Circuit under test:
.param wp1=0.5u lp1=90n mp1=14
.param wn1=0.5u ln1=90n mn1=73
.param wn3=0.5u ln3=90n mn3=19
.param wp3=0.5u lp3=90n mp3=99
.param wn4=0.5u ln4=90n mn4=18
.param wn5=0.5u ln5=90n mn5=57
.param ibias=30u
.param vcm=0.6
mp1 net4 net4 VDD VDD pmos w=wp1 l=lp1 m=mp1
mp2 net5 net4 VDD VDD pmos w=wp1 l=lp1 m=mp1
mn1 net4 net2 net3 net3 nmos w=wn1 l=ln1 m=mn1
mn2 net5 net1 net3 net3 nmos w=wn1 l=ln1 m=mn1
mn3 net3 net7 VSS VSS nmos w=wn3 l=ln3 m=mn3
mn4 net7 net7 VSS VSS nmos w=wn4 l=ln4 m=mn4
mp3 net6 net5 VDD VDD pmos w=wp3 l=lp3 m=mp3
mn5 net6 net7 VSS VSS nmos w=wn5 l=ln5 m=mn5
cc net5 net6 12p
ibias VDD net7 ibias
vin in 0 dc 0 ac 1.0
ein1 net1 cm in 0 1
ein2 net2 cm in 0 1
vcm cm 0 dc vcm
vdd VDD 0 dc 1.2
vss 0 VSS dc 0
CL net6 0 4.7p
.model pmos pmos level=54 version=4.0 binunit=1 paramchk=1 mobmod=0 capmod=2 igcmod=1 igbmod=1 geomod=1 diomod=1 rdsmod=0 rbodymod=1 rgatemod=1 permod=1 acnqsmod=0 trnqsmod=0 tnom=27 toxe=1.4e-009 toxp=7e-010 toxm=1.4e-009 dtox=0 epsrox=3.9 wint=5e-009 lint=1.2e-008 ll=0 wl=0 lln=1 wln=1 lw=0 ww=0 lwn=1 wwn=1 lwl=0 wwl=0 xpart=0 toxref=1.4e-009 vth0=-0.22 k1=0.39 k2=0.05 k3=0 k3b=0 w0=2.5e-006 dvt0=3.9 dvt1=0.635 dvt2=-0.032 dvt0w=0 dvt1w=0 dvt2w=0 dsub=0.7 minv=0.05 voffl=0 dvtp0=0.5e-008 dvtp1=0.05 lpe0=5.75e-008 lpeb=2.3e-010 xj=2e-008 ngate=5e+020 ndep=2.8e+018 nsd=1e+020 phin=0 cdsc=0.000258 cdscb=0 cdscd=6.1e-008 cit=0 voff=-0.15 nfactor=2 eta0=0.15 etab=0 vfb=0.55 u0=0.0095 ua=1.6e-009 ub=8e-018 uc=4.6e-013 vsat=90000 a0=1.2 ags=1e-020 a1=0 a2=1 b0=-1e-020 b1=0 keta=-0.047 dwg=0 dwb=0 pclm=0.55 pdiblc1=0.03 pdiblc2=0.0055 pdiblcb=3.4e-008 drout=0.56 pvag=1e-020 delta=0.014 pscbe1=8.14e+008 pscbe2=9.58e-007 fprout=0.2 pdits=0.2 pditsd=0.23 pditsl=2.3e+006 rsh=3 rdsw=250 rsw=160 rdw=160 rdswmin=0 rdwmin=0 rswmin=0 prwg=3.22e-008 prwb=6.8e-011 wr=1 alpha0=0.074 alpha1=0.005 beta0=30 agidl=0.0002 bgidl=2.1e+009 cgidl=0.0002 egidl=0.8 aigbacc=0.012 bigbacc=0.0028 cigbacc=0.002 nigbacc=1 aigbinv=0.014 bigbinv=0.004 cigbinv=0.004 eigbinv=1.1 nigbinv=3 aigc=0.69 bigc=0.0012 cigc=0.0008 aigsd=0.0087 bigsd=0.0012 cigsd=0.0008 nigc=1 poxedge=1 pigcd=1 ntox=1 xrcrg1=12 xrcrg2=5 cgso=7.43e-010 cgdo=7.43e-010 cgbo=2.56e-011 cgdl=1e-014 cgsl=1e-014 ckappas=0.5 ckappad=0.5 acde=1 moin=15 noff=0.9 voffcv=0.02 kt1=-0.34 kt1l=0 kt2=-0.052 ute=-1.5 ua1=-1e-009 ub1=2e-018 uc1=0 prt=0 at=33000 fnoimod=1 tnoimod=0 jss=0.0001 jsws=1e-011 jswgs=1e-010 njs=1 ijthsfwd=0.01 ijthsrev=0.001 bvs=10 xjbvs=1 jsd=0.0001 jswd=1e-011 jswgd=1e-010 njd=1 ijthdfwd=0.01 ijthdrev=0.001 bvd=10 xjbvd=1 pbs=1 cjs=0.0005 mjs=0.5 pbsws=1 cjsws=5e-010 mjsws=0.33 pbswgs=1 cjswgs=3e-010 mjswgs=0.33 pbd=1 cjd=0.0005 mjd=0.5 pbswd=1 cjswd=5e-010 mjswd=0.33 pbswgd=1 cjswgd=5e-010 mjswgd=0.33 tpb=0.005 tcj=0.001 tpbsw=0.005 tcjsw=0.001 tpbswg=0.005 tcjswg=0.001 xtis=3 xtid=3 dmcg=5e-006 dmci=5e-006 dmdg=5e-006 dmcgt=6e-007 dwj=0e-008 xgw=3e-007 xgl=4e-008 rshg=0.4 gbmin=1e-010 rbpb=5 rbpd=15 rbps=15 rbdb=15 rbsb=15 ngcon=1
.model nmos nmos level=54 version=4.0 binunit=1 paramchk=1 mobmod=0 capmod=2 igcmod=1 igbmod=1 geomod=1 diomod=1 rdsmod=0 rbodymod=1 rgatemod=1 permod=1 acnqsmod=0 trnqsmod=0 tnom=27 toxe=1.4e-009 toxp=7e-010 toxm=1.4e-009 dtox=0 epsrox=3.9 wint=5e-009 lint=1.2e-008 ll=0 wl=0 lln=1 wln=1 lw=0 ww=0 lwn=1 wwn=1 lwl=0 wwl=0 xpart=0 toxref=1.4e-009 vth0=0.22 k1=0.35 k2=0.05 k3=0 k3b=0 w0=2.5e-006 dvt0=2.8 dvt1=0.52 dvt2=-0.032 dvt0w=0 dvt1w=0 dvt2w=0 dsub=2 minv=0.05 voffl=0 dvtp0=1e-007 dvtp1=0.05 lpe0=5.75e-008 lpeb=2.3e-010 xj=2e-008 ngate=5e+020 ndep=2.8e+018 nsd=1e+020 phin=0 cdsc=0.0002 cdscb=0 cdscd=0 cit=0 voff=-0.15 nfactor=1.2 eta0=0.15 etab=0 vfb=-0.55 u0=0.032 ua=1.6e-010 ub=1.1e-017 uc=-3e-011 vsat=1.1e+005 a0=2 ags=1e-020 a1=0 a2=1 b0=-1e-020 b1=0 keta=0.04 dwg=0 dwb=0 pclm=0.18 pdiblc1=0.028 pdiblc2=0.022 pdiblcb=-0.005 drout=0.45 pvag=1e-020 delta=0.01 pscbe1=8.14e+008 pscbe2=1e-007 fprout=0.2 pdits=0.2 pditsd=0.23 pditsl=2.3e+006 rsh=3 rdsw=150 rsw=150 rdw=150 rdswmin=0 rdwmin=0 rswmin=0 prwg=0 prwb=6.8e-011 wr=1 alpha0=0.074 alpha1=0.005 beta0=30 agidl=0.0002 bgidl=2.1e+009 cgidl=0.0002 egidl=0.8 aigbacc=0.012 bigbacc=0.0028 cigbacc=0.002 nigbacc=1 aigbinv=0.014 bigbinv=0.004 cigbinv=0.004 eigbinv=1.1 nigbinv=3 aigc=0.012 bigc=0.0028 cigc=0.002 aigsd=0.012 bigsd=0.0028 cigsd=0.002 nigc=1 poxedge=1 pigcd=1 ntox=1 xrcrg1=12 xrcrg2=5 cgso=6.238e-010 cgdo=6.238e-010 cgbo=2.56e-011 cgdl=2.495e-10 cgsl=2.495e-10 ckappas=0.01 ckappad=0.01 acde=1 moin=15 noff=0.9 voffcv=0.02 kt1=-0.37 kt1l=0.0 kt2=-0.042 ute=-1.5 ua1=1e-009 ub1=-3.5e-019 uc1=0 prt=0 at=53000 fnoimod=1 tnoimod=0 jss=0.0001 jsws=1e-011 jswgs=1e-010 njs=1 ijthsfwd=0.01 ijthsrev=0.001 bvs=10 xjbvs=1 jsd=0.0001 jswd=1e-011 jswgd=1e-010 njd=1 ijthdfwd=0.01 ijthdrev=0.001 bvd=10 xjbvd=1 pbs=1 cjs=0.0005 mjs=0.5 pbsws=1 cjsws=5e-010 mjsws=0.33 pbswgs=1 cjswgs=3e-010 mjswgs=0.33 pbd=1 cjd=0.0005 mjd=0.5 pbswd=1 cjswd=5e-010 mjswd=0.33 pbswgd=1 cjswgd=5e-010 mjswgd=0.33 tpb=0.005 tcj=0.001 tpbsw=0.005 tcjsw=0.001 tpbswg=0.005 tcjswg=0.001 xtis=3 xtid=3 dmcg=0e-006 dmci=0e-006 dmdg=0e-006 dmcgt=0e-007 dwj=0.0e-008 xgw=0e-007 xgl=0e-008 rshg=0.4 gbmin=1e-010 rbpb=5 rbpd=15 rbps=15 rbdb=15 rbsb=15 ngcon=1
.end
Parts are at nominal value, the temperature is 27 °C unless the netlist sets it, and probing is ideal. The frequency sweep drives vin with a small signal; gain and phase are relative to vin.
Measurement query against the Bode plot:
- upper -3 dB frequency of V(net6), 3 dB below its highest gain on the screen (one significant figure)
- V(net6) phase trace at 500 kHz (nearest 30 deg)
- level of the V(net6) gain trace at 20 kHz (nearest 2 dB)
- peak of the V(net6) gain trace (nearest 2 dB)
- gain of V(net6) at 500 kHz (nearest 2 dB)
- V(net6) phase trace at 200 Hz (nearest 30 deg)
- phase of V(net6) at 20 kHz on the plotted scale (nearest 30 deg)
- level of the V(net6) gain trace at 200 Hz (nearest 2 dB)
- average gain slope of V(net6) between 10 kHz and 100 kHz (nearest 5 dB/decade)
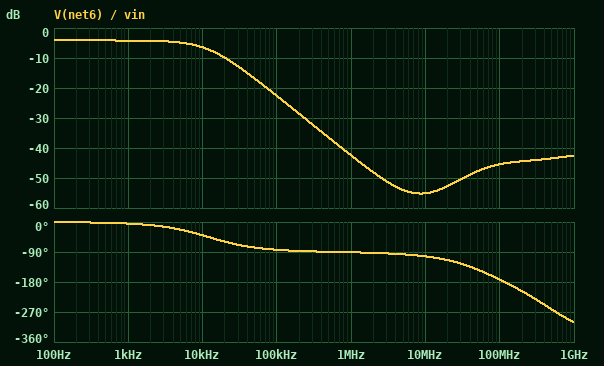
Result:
10 kHz
-90 deg
-10 dB
-4 dB
-36 dB
0 deg
-60 deg
-4 dB
-15 dB/decade
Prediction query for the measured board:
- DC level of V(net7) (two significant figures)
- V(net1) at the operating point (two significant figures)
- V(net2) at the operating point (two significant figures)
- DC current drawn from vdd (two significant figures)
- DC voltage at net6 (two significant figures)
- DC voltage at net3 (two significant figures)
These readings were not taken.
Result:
350 mV
600 mV
600 mV
180 µA
690 mV
350 mV
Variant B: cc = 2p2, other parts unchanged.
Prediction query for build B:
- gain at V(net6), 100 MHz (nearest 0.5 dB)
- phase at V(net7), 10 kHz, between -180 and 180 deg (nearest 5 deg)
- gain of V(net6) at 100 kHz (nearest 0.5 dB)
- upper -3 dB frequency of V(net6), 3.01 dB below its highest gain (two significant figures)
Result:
-43.5 dB
-10 deg
-9.5 dB
63 kHz
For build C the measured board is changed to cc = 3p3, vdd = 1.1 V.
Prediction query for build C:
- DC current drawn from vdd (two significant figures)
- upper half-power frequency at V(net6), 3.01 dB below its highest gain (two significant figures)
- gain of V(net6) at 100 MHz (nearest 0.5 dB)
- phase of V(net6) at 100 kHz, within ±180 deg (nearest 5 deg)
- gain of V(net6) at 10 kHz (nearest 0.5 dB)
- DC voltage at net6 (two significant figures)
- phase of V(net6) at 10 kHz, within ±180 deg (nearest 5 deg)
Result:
170 µA
44 kHz
-44.0 dB
-65 deg
-4.0 dB
650 mV
-15 deg
